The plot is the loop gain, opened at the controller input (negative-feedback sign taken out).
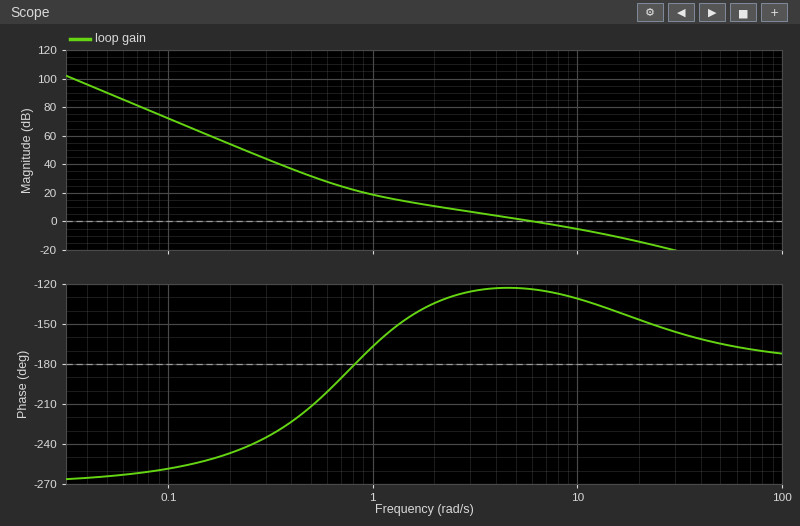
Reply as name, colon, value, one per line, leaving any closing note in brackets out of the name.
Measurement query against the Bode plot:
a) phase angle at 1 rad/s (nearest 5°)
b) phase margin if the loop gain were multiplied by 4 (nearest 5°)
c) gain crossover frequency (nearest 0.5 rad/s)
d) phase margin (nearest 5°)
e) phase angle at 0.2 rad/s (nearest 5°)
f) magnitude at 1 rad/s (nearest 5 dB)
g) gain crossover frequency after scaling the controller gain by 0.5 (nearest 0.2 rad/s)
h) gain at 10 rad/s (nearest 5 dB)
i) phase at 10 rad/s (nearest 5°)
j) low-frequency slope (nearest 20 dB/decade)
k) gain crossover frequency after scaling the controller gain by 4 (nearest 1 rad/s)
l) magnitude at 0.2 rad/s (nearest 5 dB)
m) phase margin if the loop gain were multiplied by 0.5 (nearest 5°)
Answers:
phase angle at 1 rad/s: -165°
phase margin if the loop gain were multiplied by 4: 35°
gain crossover frequency: 6.0 rad/s
phase margin: 55°
phase angle at 0.2 rad/s: -245°
magnitude at 1 rad/s: 20 dB
gain crossover frequency after scaling the controller gain by 0.5: 3.2 rad/s
gain at 10 rad/s: -5 dB
phase at 10 rad/s: -130°
low-frequency slope: -60 dB/decade
gain crossover frequency after scaling the controller gain by 4: 17 rad/s
magnitude at 0.2 rad/s: 55 dB
phase margin if the loop gain were multiplied by 0.5: 55°
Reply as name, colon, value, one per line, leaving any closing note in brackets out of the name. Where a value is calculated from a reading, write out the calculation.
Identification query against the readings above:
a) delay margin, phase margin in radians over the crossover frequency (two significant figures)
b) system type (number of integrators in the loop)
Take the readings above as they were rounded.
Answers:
delay margin, phase margin in radians over the crossover frequency: 55 × π / 180 / 6 = 0.16 s
system type: 3
